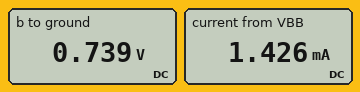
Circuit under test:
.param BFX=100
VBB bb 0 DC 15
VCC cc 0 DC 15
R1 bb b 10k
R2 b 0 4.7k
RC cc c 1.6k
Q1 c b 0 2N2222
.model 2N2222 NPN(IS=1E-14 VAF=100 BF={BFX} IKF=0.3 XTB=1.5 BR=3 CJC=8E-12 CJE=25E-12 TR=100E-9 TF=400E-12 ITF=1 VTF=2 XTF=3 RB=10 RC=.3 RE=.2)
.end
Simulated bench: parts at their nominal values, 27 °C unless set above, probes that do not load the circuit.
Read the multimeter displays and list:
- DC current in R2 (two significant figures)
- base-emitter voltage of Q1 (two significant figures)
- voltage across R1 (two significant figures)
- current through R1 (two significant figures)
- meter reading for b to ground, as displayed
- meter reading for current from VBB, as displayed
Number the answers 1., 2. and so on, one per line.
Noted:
1. 160 µA
2. 740 mV
3. 14 V
4. 1.4 mA
5. 0.739 V
6. 1.426 mA
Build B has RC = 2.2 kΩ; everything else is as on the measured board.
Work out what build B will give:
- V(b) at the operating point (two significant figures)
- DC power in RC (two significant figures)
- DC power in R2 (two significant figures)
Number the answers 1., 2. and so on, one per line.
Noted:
1. 730 mV
2. 100 mW
3. 110 µW
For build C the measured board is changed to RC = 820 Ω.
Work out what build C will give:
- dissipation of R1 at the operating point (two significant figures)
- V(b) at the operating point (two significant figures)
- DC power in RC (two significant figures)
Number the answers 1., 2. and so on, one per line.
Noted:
1. 20 mW
2. 750 mV
3. 270 mW
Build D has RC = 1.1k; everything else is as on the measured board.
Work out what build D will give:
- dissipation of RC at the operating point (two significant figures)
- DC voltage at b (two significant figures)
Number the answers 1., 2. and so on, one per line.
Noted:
1. 200 mW
2. 750 mV
